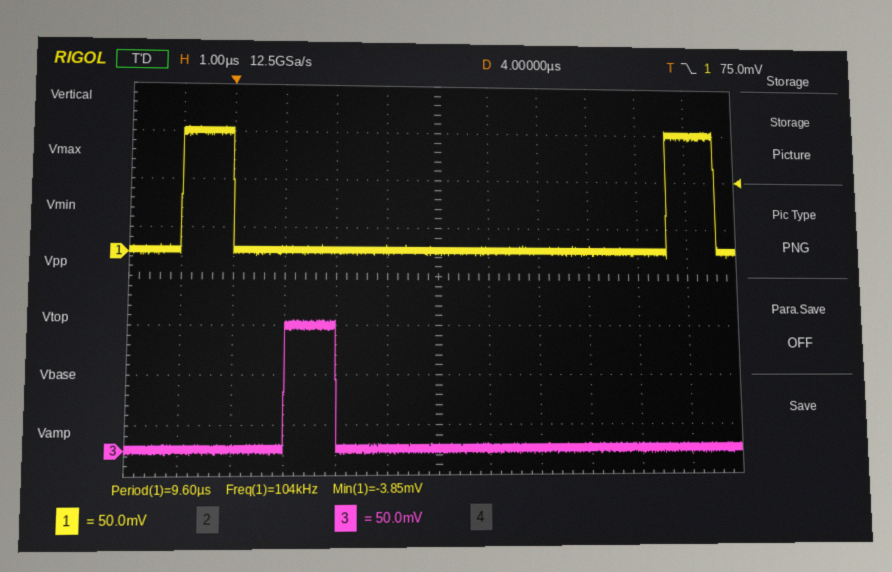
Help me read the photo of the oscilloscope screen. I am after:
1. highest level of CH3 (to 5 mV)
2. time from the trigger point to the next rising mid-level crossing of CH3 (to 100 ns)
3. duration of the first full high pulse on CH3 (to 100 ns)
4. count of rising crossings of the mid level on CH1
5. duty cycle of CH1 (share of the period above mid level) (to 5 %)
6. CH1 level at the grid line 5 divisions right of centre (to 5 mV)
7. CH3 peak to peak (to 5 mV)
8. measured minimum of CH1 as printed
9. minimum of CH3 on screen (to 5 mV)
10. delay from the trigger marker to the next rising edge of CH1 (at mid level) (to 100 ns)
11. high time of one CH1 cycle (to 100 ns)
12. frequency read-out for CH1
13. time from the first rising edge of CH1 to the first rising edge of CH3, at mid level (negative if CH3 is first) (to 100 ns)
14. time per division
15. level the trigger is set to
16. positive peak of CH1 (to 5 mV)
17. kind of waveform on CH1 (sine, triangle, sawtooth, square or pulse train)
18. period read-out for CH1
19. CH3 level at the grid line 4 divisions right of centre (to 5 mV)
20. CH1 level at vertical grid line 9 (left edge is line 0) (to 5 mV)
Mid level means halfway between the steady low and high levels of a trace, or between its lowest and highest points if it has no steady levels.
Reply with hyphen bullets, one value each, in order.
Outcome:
- 130 mV
- 1.0 µs
- 1.0 µs
- 2
- 10 %
- 125 mV
- 135 mV
- -3.85 mV
- -5 mV
- 8.6 µs
- 1.0 µs
- 104 kHz
- +2.0 µs
- 1 µs
- 75.0 mV
- 130 mV
- pulse train
- 9.60 µs
- 0 mV
- 5 mV
